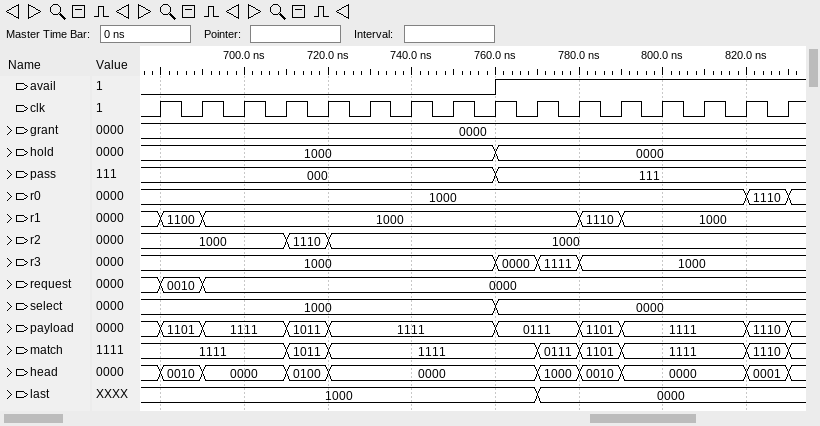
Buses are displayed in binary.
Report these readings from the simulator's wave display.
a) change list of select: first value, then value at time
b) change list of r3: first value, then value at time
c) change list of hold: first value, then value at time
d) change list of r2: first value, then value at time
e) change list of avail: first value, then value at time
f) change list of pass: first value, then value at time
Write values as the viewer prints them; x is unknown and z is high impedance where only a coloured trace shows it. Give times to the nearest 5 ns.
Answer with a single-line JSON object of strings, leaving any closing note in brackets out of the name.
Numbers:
{"change list of select: first value, then value at time": "1000, 0000 at 760 ns", "change list of r3: first value, then value at time": "1000, 0000 at 760 ns, 1111 at 770 ns, 1000 at 780 ns", "change list of hold: first value, then value at time": "1000, 0000 at 760 ns", "change list of r2: first value, then value at time": "1000, 1110 at 710 ns, 1000 at 720 ns", "change list of avail: first value, then value at time": "0, 1 at 760 ns", "change list of pass: first value, then value at time": "000, 111 at 760 ns"}
